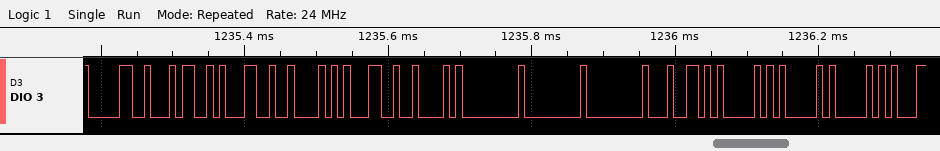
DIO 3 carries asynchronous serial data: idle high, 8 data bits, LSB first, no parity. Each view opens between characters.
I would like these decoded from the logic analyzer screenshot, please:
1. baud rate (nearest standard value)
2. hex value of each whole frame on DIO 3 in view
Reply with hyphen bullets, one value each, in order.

- 115200 baud
- 30, 34, 31, 42, 31, 42, 00, 00, 00, 64, 41, 41, 50
